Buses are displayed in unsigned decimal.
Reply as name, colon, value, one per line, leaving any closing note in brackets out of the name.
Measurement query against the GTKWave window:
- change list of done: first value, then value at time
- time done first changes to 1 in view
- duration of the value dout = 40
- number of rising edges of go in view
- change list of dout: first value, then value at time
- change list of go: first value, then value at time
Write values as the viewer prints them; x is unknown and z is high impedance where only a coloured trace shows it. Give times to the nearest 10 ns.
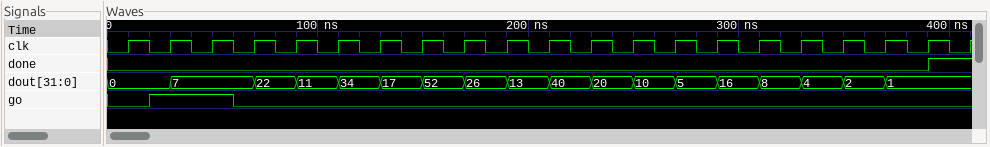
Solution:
change list of done: first value, then value at time: 0, 1 at 390 ns
time done first changes to 1 in view: 390 ns
duration of the value dout = 40: 20 ns
number of rising edges of go in view: 1
change list of dout: first value, then value at time: 0, 7 at 30 ns, 22 at 70 ns, 11 at 90 ns, 34 at 110 ns, 17 at 130 ns, 52 at 150 ns, 26 at 170 ns, 13 at 190 ns, 40 at 210 ns, 20 at 230 ns, 10 at 250 ns, 5 at 270 ns, 16 at 290 ns, 8 at 310 ns, 4 at 330 ns, 2 at 350 ns, 1 at 370 ns
change list of go: first value, then value at time: 0, 1 at 20 ns, 0 at 60 ns
